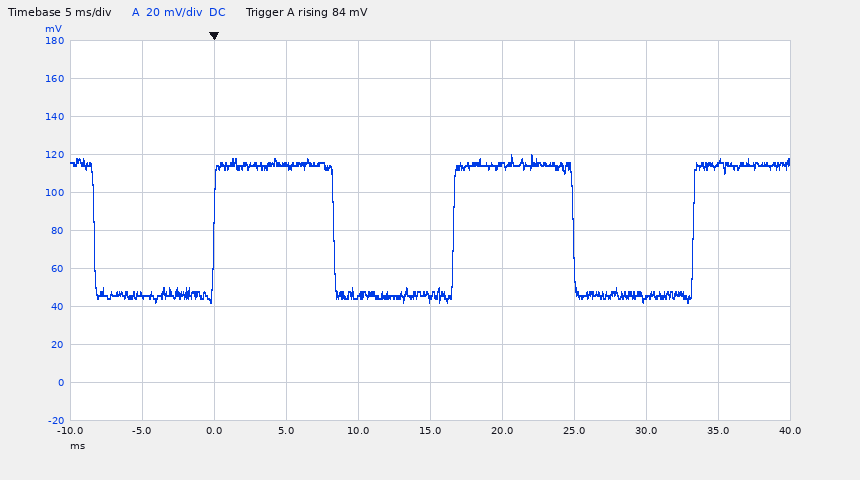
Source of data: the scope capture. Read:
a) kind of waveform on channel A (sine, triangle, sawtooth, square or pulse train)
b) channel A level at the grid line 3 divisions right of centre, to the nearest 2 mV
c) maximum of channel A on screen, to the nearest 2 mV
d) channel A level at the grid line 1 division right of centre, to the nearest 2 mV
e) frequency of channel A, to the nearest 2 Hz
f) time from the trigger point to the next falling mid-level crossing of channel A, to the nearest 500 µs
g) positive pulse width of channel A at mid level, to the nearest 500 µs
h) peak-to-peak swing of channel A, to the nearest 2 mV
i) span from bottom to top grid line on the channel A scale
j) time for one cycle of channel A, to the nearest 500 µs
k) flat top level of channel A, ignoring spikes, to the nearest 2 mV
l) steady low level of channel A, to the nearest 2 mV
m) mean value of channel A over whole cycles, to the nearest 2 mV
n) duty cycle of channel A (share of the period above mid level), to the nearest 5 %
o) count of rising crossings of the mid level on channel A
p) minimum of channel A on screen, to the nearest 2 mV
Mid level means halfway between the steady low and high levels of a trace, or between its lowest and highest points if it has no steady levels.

square
44 mV
120 mV
114 mV
60 Hz
8.5 ms
8.5 ms
78 mV
200 mV
16.5 ms
114 mV
46 mV
80 mV
50 %
3
42 mV
